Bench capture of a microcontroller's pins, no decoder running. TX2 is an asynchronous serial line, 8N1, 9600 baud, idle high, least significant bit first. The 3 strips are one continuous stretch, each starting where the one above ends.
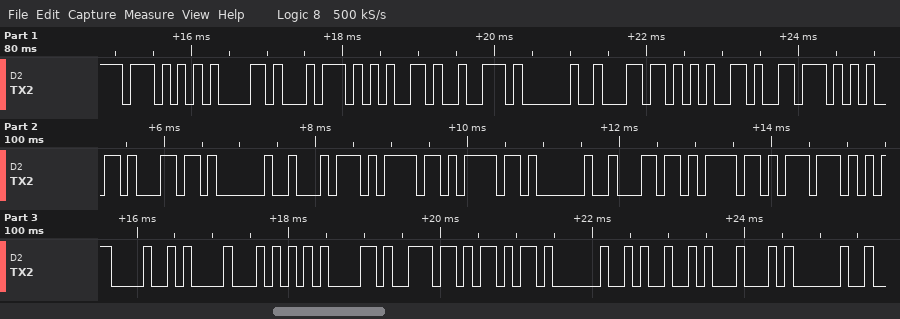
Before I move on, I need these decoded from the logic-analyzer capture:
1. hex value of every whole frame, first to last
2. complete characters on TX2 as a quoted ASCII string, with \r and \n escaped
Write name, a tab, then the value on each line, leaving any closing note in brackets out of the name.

hex value of every whole frame, first to last	57 61 74 65 72 20 6C 65 76 65 6C 20 74 6F 6F 20 6C 6F 77 0D 0A 54 61 6E 6B 20 49 44 20
complete characters on TX2 as a quoted ASCII string, with \r and \n escaped	"Water level too low\r\nTank ID "
